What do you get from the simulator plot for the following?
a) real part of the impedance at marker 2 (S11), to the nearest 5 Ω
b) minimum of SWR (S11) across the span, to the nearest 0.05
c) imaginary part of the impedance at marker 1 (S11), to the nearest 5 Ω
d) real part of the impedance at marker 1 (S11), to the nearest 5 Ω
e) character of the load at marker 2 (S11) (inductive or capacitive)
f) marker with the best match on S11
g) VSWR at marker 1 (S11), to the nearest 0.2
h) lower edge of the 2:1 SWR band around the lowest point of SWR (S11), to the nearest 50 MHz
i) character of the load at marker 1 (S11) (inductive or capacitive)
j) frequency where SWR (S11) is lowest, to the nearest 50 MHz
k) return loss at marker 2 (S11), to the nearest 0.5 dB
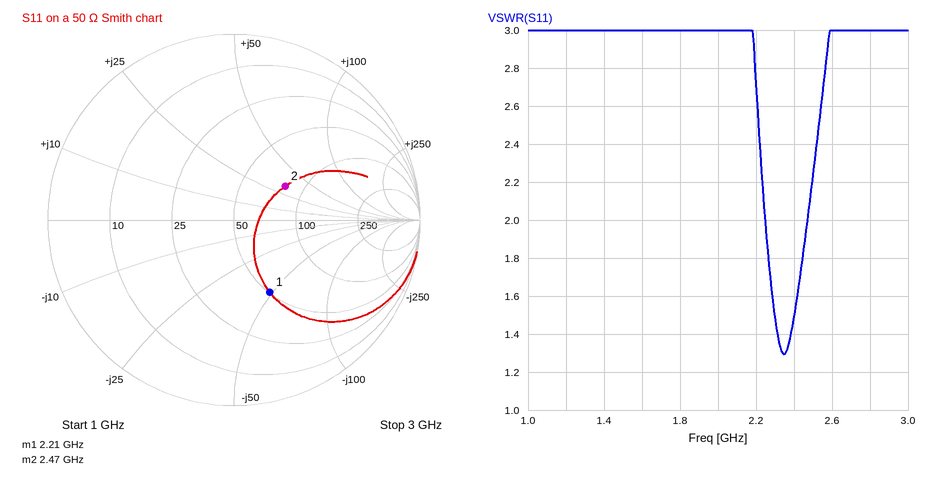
80 Ω
1.30
-50 Ω
50 Ω
inductive
marker 2
2.6
2.25 GHz
capacitive
2.35 GHz
9.5 dB
